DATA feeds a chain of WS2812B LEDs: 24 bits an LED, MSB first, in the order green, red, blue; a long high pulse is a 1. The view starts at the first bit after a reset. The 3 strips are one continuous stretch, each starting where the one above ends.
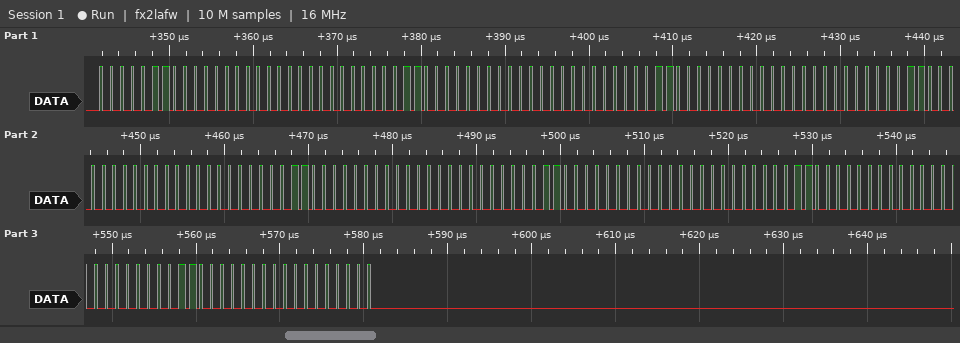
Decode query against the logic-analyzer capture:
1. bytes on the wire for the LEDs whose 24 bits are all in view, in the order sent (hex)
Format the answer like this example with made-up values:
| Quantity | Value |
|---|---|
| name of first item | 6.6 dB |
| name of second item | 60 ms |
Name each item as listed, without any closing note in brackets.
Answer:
| Quantity | Value |
|---|---|
| bytes on the wire for the LEDs whose 24 bits are all in view, in the order sent | 06 00 00 06 00 00 06 00 00 06 00 00 06 00 00 06 00 00 06 00 00 06 00 00 |
